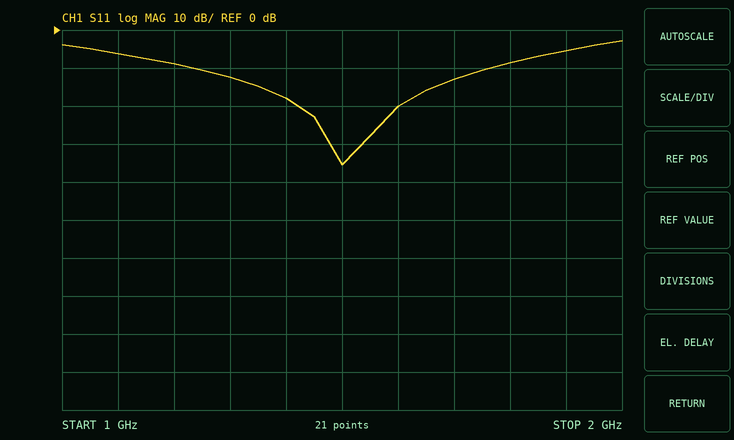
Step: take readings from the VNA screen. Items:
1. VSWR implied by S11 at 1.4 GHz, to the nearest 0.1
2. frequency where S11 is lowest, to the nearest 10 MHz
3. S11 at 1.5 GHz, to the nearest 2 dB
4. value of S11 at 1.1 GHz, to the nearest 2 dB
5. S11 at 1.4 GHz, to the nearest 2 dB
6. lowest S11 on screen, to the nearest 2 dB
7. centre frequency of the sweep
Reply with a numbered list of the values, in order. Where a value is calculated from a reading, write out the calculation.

1. |Γ| = 10^(-18/20) = 0.1259; VSWR = (1 + 0.1259)/(1 − 0.1259) ≈ 1.3
2. 1.50 GHz
3. -36 dB
4. -6 dB
5. -18 dB
6. -36 dB
7. 1.5 GHz
